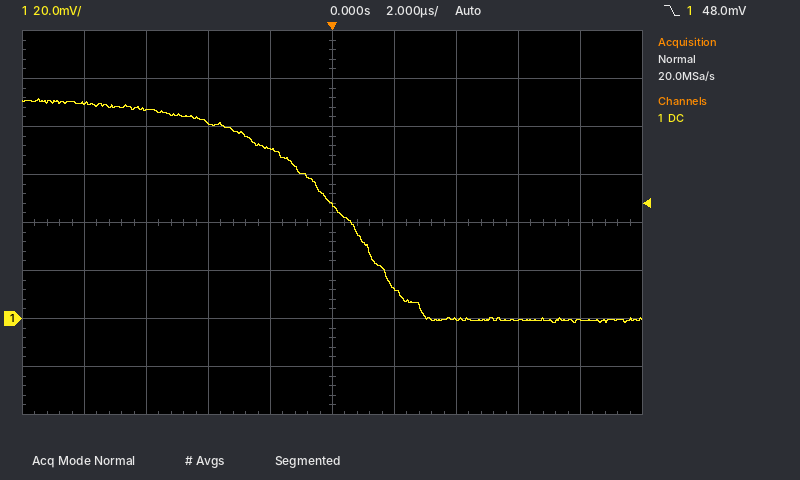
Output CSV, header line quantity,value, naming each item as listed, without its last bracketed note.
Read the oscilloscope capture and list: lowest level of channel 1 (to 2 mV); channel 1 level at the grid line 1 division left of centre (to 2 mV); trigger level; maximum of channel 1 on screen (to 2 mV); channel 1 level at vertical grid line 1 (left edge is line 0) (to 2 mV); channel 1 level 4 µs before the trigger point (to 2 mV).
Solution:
quantity,value
lowest level of channel 1,-2 mV
channel 1 level at the grid line 1 division left of centre,70 mV
trigger level,48.0 mV
maximum of channel 1 on screen,92 mV
channel 1 level at vertical grid line 1 (left edge is line 0),90 mV
channel 1 level 4 µs before the trigger point,82 mV
